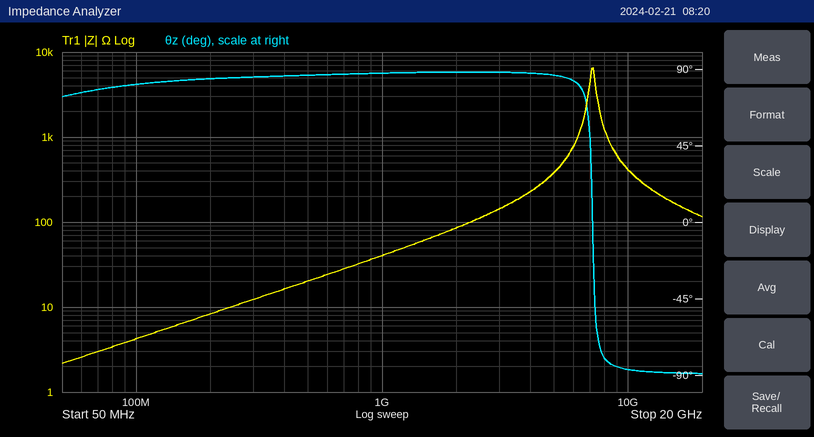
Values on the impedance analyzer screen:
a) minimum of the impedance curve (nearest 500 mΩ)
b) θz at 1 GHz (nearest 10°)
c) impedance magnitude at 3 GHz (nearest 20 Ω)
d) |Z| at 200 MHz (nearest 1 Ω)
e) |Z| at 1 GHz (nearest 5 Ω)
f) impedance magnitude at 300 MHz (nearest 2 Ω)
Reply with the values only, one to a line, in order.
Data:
2.0 Ω
90°
140 Ω
8 Ω
40 Ω
12 Ω
